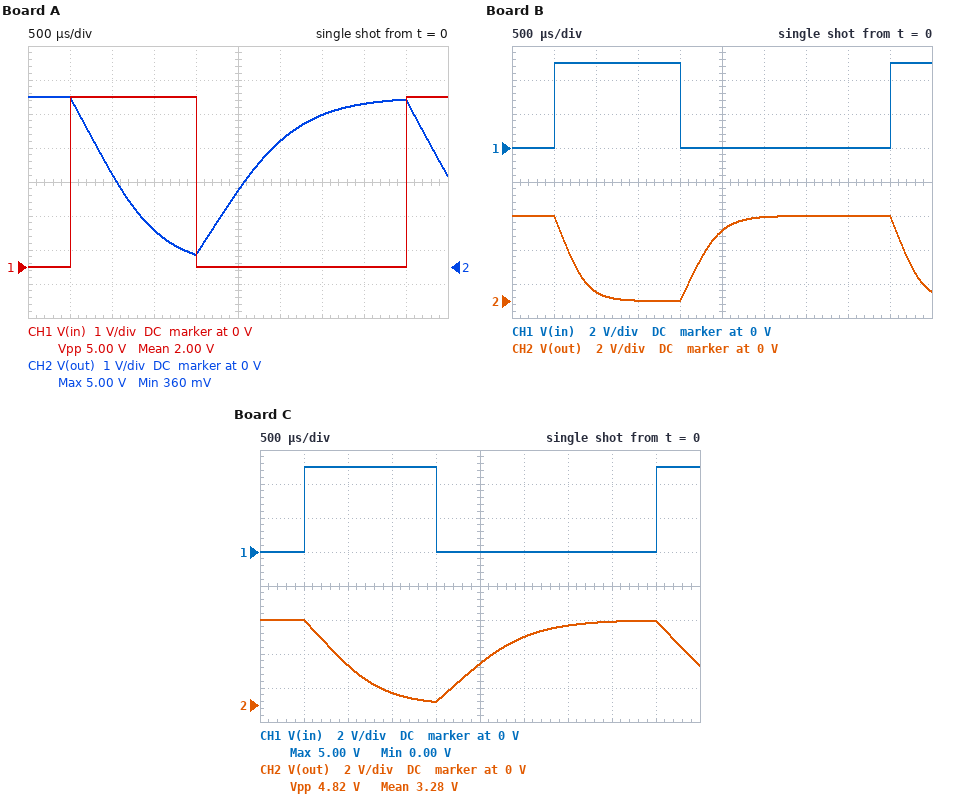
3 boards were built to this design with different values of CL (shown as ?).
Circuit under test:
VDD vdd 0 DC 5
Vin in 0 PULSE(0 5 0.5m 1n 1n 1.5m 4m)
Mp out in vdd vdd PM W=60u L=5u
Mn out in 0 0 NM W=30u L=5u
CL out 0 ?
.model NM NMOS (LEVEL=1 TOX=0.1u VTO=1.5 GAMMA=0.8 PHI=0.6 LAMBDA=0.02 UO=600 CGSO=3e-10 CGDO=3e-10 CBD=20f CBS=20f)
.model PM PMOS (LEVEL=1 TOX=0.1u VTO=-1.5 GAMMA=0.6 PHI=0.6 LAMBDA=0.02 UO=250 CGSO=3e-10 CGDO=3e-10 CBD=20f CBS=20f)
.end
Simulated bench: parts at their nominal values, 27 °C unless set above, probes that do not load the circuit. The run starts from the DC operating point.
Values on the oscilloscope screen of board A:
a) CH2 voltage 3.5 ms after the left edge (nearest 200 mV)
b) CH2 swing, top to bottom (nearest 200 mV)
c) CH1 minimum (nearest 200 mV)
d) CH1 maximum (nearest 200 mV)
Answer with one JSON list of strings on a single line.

["4.4 V", "4.6 V", "0 V", "5.0 V"]
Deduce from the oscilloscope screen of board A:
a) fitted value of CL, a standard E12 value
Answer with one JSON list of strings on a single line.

["180 nF"]
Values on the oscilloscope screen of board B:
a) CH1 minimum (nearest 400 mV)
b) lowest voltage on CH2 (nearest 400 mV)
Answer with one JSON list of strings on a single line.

["0 V", "0 V"]
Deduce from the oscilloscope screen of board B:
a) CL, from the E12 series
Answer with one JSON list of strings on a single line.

["68 nF"]
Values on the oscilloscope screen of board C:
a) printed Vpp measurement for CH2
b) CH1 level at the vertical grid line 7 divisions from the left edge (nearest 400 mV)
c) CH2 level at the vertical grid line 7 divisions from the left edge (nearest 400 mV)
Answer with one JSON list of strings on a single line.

["4.82 V", "0 V", "4.8 V"]
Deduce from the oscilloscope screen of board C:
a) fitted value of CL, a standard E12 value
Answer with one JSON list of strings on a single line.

["150 nF"]
